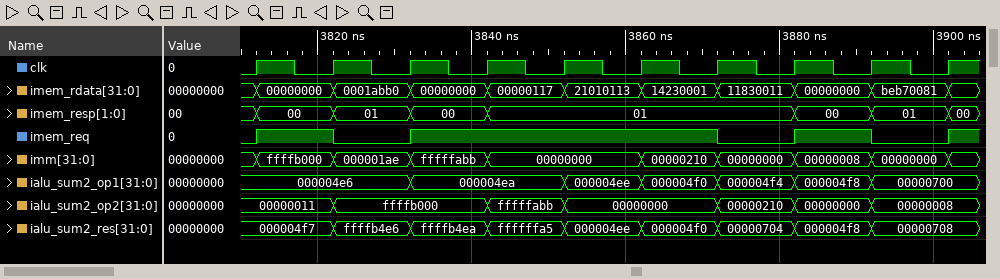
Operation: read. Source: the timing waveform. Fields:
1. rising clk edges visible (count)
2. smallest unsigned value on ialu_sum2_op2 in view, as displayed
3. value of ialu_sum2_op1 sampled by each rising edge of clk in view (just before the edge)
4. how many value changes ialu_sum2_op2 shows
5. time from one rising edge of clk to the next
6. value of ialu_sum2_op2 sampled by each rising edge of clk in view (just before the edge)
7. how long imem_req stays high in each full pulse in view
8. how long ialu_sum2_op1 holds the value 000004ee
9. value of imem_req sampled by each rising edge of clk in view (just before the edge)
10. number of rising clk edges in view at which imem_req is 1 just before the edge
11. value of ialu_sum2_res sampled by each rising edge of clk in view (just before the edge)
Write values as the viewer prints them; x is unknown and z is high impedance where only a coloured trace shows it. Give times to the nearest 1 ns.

10
00000000
000004e6, 000004e6, 000004e6, 000004ea, 000004ea, 000004ee, 000004f0, 000004f4, 000004f8, 00000700
6
10 ns
00000011, 00000011, ffffb000, ffffb000, fffffabb, 00000000, 00000000, 00000210, 00000000, 00000008
10 ns, 40 ns, 10 ns
10 ns
0 1 0 1 1 1 1 0 1 0
6
000004f7, 000004f7, ffffb4e6, ffffb4ea, ffffffa5, 000004ee, 000004f0, 00000704, 000004f8, 00000708
